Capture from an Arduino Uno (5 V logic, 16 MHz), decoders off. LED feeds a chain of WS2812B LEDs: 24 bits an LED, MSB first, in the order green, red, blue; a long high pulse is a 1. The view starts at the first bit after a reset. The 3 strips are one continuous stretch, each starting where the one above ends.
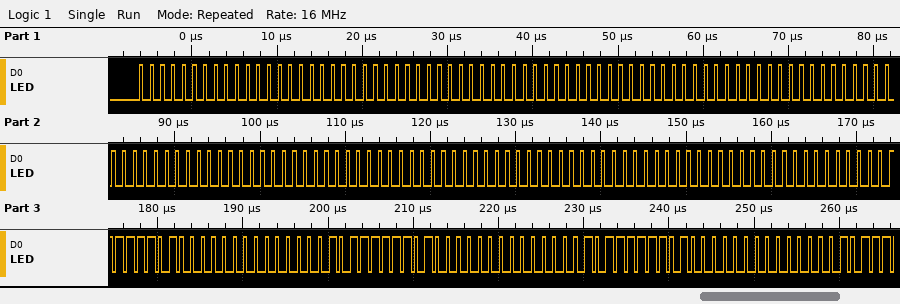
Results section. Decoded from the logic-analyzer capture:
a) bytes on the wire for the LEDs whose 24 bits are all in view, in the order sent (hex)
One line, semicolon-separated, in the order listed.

00 00 00 00 00 00 00 00 00 00 00 00 00 00 00 00 00 00 FA 00 05 FA 00 05 FA 00 05
